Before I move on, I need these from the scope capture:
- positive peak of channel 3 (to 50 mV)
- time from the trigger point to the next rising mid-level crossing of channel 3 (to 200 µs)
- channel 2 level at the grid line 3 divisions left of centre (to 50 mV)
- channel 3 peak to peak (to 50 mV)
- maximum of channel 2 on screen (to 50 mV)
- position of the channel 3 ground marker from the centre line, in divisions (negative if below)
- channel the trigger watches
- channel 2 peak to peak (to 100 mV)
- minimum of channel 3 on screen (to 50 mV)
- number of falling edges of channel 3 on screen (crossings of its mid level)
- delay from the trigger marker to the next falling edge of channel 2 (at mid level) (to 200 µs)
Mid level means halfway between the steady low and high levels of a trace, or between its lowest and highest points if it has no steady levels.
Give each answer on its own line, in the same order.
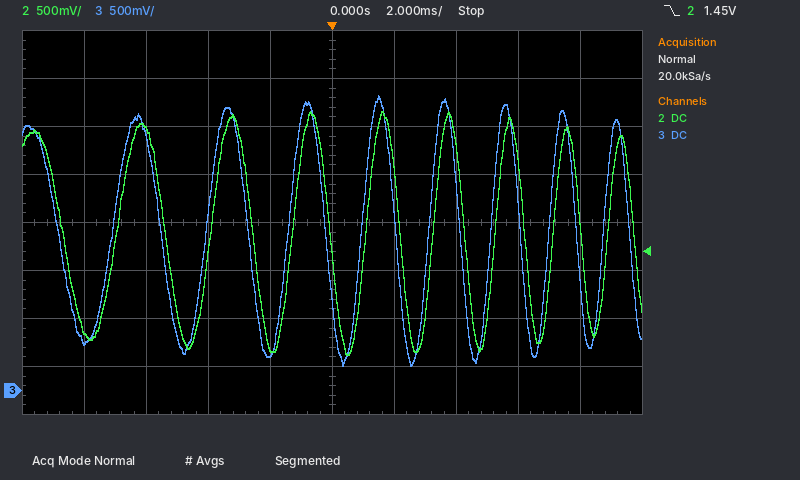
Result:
3.05 V
1.0 ms
2.75 V
2.80 V
2.90 V
-3.5 div
channel 2
2.50 V
250 mV
9
2.2 ms
